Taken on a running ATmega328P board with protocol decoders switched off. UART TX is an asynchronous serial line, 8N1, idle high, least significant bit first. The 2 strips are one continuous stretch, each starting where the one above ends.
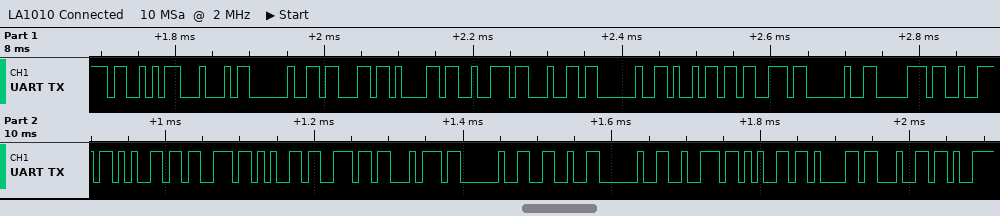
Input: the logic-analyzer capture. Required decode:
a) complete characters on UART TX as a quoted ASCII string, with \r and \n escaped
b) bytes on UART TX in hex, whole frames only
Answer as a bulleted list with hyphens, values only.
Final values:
- "SD card is present & read"
- 53 44 20 63 61 72 64 20 69 73 20 70 72 65 73 65 6E 74 20 26 20 72 65 61 64
